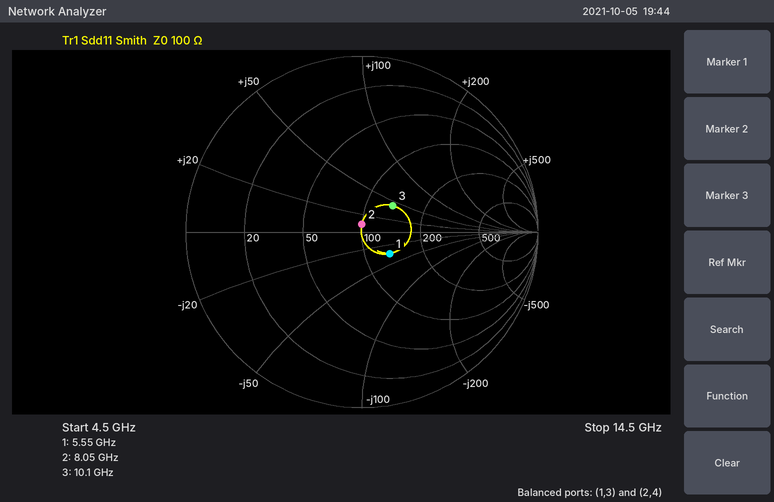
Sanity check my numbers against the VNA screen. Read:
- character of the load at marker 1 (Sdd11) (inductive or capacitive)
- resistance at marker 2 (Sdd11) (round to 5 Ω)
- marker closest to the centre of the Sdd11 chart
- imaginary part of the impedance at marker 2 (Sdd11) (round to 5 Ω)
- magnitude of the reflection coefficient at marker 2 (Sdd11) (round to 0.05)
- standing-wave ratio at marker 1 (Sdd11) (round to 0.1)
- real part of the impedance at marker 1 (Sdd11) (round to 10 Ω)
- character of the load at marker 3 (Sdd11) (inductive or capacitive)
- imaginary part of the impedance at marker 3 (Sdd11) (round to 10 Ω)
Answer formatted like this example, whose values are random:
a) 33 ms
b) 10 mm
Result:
a) capacitive
b) 100 Ω
c) marker 2
d) +10 Ω
e) 0.05
f) 1.5
g) 130 Ω
h) inductive
i) +40 Ω
